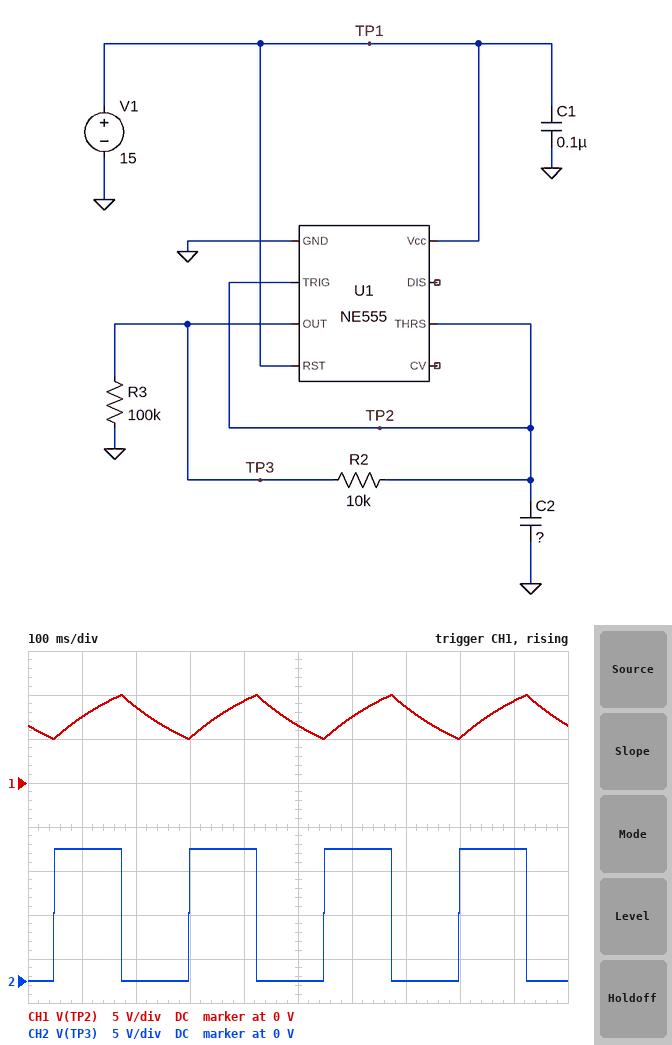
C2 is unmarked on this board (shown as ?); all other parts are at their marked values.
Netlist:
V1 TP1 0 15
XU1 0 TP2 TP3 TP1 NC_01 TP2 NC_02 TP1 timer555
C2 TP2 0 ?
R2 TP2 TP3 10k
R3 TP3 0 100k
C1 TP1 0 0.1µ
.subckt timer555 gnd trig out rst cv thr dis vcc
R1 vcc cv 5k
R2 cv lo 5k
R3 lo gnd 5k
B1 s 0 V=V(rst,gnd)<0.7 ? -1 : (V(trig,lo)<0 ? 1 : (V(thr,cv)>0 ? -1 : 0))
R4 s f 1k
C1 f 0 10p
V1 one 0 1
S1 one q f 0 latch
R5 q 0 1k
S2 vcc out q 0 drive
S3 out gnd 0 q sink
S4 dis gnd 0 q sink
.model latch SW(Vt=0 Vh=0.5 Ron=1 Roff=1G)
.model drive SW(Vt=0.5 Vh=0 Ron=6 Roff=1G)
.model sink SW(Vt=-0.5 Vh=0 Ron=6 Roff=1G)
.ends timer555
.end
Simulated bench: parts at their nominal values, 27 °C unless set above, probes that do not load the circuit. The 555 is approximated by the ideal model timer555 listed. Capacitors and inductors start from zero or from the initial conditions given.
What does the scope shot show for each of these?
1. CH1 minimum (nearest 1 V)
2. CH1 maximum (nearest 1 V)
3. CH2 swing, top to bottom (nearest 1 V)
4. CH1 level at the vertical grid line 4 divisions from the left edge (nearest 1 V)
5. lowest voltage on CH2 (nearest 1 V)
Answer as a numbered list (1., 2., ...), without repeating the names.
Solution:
1. 5 V
2. 10 V
3. 15 V
4. 9 V
5. 0 V
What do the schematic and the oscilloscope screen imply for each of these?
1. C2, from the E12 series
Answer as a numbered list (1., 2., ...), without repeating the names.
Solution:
1. 18 µF
